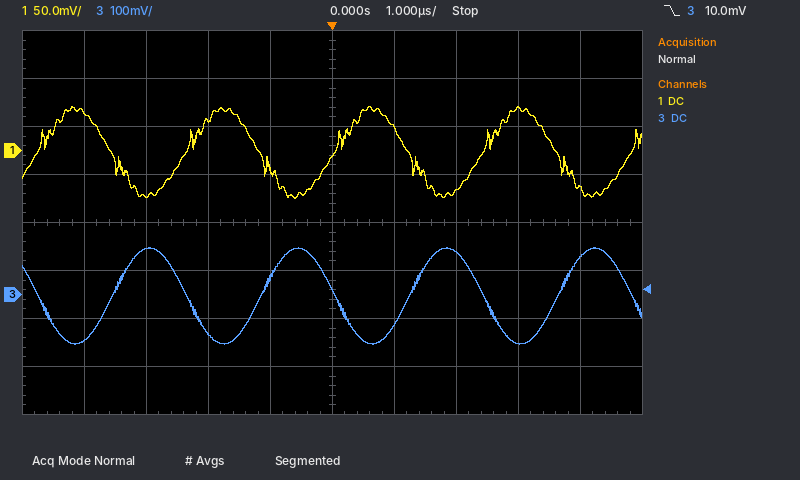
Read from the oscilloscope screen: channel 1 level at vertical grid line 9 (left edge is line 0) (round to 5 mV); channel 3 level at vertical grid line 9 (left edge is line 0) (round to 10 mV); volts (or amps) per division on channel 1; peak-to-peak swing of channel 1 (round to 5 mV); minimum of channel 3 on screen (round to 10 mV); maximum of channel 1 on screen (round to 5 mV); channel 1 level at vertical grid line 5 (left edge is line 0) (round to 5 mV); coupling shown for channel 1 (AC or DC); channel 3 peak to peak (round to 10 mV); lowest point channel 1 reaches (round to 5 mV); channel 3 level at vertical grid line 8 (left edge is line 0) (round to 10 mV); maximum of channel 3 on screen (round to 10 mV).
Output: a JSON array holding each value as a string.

["-40 mV", "80 mV", "50 mV", "95 mV", "-100 mV", "45 mV", "-5 mV", "DC", "200 mV", "-50 mV", "-100 mV", "100 mV"]
